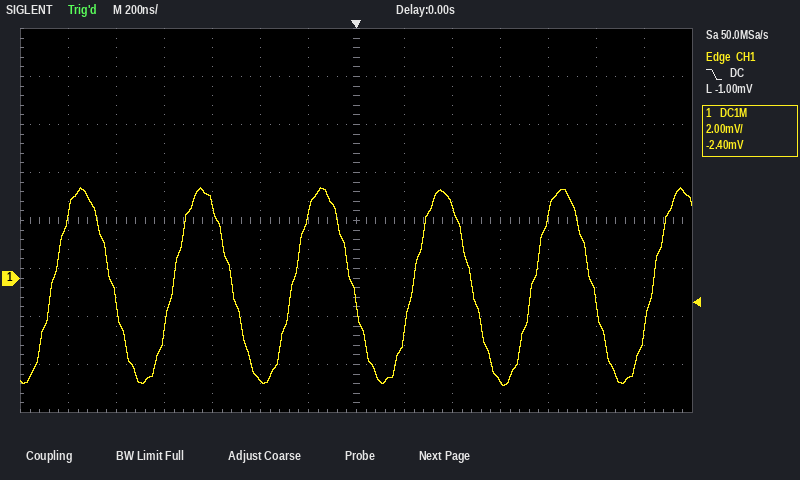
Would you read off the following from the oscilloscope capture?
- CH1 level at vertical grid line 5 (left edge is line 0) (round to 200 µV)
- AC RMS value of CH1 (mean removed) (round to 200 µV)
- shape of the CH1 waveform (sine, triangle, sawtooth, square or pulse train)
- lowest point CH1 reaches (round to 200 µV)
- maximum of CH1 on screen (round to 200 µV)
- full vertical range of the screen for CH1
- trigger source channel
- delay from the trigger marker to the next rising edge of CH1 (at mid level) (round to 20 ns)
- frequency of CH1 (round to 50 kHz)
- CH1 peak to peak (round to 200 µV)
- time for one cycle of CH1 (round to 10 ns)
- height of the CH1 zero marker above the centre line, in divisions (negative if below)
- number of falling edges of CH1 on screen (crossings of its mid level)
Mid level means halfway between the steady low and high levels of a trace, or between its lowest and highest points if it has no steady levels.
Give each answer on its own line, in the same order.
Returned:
-4.2 mV
2.8 mV
sine
-4.4 mV
3.8 mV
16 mV
CH1
240 ns
2.00 MHz
8.2 mV
500 ns
-1.2 div
5
